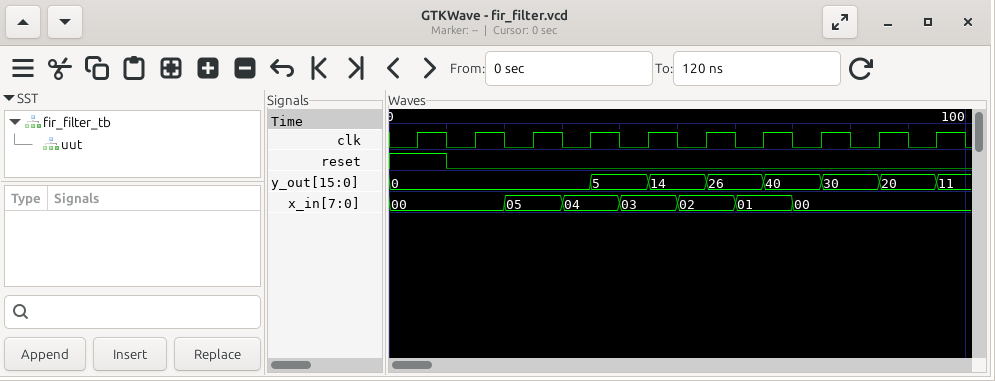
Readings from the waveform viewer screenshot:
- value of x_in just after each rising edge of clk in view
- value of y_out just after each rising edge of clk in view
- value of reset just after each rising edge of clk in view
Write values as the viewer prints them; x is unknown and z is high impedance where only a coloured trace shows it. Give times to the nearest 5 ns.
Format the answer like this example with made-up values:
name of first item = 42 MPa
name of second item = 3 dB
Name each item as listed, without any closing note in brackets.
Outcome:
value of x_in just after each rising edge of clk in view = 00, 00, 05, 04, 03, 02, 01, 00, 00, 00
value of y_out just after each rising edge of clk in view = 0, 0, 0, 5, 14, 26, 40, 30, 20, 11
value of reset just after each rising edge of clk in view = 1 0 0 0 0 0 0 0 0 0
